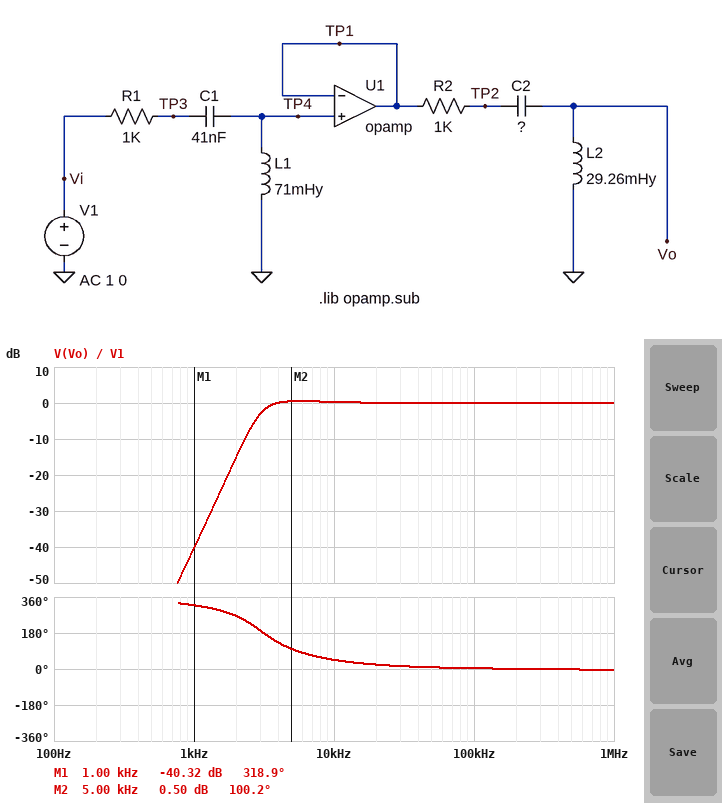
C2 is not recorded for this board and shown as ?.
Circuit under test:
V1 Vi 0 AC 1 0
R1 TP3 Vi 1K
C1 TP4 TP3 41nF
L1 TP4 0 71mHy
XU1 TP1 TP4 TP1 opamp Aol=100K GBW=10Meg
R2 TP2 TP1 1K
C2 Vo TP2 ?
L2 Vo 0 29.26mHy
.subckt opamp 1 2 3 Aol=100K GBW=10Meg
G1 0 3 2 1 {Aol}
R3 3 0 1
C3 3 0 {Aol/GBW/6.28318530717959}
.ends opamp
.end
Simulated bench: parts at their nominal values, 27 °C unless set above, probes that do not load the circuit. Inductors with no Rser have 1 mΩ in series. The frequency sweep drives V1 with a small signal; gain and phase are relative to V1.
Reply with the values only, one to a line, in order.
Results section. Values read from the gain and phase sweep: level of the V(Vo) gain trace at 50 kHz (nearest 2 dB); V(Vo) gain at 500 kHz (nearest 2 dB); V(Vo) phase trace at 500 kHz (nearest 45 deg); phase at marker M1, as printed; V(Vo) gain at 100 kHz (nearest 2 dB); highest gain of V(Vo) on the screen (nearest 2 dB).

0 dB
0 dB
0 deg
318.9 deg
0 dB
0 dB
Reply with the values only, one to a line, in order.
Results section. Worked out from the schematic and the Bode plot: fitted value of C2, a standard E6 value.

68 nF
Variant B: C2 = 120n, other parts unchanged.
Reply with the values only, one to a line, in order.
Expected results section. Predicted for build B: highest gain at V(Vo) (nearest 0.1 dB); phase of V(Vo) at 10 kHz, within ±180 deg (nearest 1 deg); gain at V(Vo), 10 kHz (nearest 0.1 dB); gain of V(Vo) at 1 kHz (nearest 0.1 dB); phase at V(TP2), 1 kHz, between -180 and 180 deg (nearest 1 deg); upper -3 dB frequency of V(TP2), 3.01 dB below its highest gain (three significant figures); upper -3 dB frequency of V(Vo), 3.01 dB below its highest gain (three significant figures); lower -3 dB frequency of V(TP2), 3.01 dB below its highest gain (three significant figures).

0 dB
44 deg
-0.1 dB
-36.4 dB
123 deg
10.0 MHz
10.0 MHz
5.13 kHz
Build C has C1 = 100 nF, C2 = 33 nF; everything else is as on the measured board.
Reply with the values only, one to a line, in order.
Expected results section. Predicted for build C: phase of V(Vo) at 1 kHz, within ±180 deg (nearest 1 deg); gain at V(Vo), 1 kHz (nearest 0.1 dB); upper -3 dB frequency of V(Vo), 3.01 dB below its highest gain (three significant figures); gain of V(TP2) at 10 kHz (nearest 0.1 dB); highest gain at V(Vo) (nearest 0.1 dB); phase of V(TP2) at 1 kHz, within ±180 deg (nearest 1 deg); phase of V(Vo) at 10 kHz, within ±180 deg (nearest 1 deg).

-53 deg
-38.9 dB
7.53 MHz
-1.8 dB
1.1 dB
127 deg
49 deg
